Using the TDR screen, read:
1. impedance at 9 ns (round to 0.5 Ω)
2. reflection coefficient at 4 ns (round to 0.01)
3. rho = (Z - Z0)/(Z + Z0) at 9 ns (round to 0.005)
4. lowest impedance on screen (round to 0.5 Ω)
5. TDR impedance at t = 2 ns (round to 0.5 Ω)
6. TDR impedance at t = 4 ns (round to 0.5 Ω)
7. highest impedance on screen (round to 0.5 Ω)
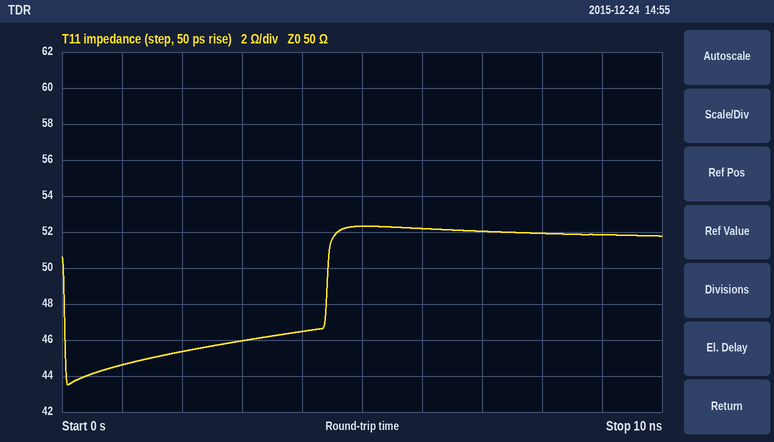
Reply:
52.0 Ω
-0.04
+0.020
43.5 Ω
45.5 Ω
46.5 Ω
52.5 Ω
